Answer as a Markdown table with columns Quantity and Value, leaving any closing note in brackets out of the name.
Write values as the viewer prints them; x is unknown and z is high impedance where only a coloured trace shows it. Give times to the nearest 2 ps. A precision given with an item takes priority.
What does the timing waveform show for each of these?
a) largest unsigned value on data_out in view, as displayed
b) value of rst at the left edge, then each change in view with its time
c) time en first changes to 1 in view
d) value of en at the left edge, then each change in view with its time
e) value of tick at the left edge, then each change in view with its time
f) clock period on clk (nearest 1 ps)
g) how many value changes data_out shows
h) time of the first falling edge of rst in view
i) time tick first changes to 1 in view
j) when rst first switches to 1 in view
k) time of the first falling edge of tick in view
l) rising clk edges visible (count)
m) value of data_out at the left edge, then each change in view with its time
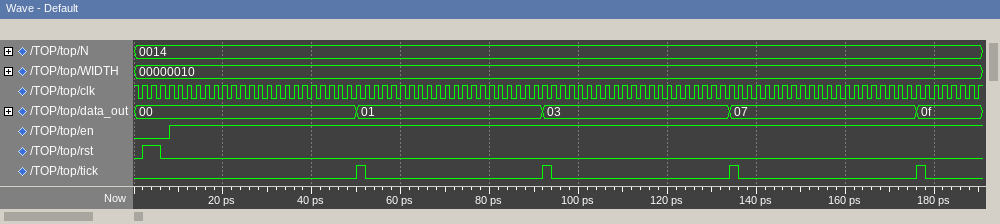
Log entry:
| Quantity | Value |
|---|---|
| largest unsigned value on data_out in view, as displayed | 0f |
| value of rst at the left edge, then each change in view with its time | 0, 1 at 2 ps, 0 at 6 ps |
| time en first changes to 1 in view | 8 ps |
| value of en at the left edge, then each change in view with its time | 0, 1 at 8 ps |
| value of tick at the left edge, then each change in view with its time | 0, 1 at 50 ps, 0 at 52 ps, 1 at 92 ps, 0 at 94 ps, 1 at 134 ps, 0 at 136 ps, 1 at 176 ps, 0 at 178 ps |
| clock period on clk | 2 ps |
| how many value changes data_out shows | 4 |
| time of the first falling edge of rst in view | 6 ps |
| time tick first changes to 1 in view | 50 ps |
| when rst first switches to 1 in view | 2 ps |
| time of the first falling edge of tick in view | 52 ps |
| rising clk edges visible | 95 |
| value of data_out at the left edge, then each change in view with its time | 00, 01 at 50 ps, 03 at 92 ps, 07 at 134 ps, 0f at 176 ps |
